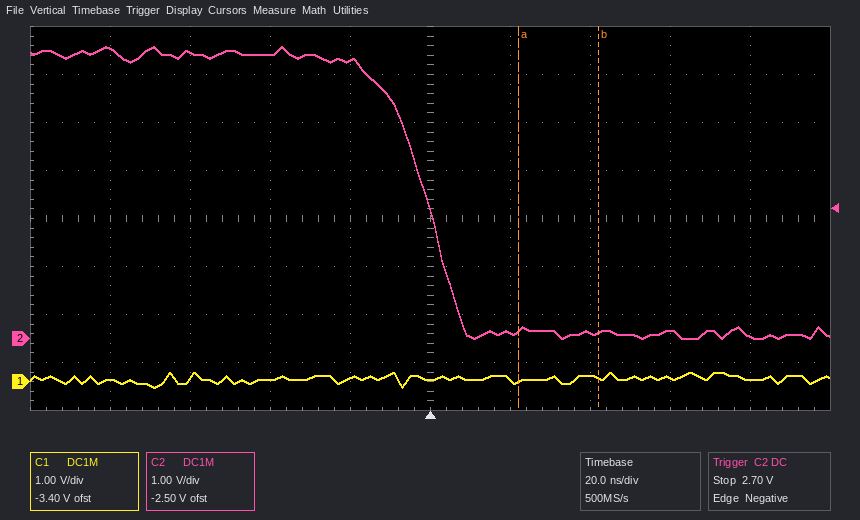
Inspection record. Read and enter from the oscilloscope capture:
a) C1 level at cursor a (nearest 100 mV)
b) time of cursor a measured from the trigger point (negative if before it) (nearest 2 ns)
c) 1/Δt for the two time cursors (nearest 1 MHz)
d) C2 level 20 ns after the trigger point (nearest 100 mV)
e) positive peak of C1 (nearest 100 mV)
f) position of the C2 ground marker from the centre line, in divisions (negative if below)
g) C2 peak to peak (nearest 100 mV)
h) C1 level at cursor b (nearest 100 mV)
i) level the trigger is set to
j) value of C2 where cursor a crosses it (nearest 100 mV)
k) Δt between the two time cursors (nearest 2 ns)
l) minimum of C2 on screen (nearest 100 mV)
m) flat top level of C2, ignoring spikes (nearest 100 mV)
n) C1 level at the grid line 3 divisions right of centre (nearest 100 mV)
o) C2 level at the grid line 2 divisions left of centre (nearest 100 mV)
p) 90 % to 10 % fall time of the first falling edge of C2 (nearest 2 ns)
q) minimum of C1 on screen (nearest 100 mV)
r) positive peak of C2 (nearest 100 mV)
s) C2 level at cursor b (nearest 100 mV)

0.0 V
+22 ns
50 MHz
100 mV
200 mV
-2.5 div
6.1 V
100 mV
2.70 V
200 mV
20 ns
0.0 V
5.9 V
100 mV
5.9 V
20 ns
-100 mV
6.1 V
100 mV
